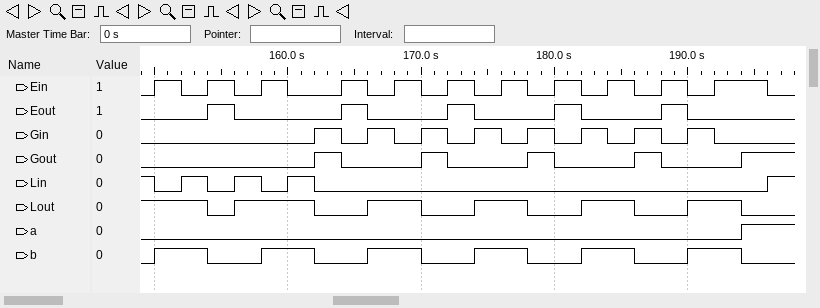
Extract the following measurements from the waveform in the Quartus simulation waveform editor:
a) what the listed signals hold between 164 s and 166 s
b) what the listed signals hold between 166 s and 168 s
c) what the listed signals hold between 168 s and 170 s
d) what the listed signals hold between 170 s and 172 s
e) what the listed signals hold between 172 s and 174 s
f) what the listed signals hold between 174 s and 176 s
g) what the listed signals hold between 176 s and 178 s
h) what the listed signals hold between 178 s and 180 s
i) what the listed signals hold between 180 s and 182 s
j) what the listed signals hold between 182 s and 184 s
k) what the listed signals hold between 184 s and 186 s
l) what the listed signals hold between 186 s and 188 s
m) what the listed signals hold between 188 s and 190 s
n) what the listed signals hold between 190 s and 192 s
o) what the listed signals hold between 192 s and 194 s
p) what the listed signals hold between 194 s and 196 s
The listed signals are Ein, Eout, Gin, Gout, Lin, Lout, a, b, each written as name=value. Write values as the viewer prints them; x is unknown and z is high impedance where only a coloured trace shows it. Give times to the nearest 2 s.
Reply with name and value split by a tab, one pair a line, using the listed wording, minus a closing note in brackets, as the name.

what the listed signals hold between 164 s and 166 s	Ein=1, Eout=1, Gin=0, Gout=0, Lin=0, Lout=0, a=0, b=0
what the listed signals hold between 166 s and 168 s	Ein=0, Eout=0, Gin=1, Gout=0, Lin=0, Lout=1, a=0, b=1
what the listed signals hold between 168 s and 170 s	Ein=1, Eout=0, Gin=0, Gout=0, Lin=0, Lout=1, a=0, b=1
what the listed signals hold between 170 s and 172 s	Ein=0, Eout=0, Gin=1, Gout=1, Lin=0, Lout=0, a=0, b=0
what the listed signals hold between 172 s and 174 s	Ein=1, Eout=1, Gin=0, Gout=0, Lin=0, Lout=0, a=0, b=0
what the listed signals hold between 174 s and 176 s	Ein=0, Eout=0, Gin=1, Gout=0, Lin=0, Lout=1, a=0, b=1
what the listed signals hold between 176 s and 178 s	Ein=1, Eout=0, Gin=0, Gout=0, Lin=0, Lout=1, a=0, b=1
what the listed signals hold between 178 s and 180 s	Ein=0, Eout=0, Gin=1, Gout=1, Lin=0, Lout=0, a=0, b=0
what the listed signals hold between 180 s and 182 s	Ein=1, Eout=1, Gin=0, Gout=0, Lin=0, Lout=0, a=0, b=0
what the listed signals hold between 182 s and 184 s	Ein=0, Eout=0, Gin=1, Gout=0, Lin=0, Lout=1, a=0, b=1
what the listed signals hold between 184 s and 186 s	Ein=1, Eout=0, Gin=0, Gout=0, Lin=0, Lout=1, a=0, b=1
what the listed signals hold between 186 s and 188 s	Ein=0, Eout=0, Gin=1, Gout=1, Lin=0, Lout=0, a=0, b=0
what the listed signals hold between 188 s and 190 s	Ein=1, Eout=1, Gin=0, Gout=0, Lin=0, Lout=0, a=0, b=0
what the listed signals hold between 190 s and 192 s	Ein=0, Eout=0, Gin=1, Gout=0, Lin=0, Lout=1, a=0, b=1
what the listed signals hold between 192 s and 194 s	Ein=1, Eout=0, Gin=0, Gout=0, Lin=0, Lout=1, a=0, b=1
what the listed signals hold between 194 s and 196 s	Ein=1, Eout=0, Gin=0, Gout=1, Lin=0, Lout=0, a=1, b=0
